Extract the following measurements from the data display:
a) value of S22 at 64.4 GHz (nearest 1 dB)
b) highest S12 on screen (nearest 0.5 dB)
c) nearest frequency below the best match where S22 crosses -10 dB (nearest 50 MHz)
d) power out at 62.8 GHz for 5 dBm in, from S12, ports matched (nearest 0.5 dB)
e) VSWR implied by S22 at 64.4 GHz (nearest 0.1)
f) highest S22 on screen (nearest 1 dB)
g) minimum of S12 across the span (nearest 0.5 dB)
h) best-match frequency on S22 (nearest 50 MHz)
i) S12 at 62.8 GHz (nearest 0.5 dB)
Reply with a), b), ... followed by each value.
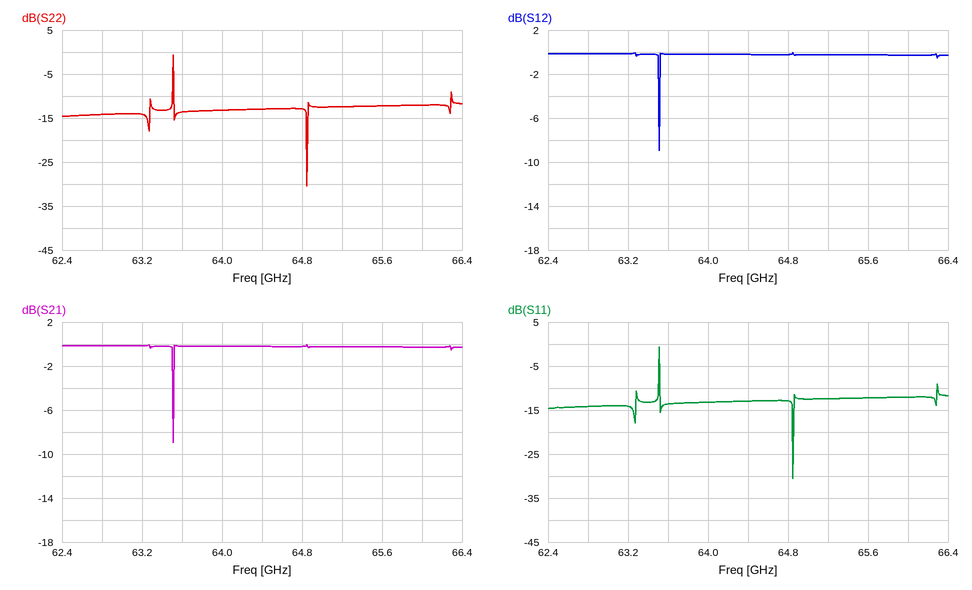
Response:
a) -13 dB
b) 0.0 dB
c) 63.50 GHz
d) 5.0 dBm
e) 1.6
f) -1 dB
g) -9.0 dB
h) 64.85 GHz
i) 0.0 dB
